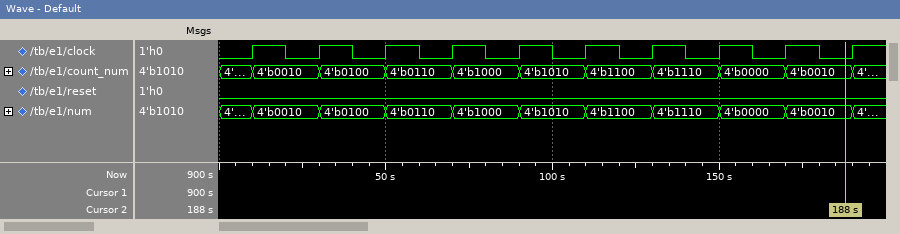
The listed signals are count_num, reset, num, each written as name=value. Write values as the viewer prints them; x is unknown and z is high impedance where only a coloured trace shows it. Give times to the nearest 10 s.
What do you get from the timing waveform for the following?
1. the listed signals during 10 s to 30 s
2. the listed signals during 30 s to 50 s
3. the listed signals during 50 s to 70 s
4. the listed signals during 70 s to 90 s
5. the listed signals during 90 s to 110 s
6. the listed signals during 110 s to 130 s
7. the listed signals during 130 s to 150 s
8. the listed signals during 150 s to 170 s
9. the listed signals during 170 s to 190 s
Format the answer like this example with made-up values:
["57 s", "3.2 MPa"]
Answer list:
["count_num=4'b0010, reset=0, num=4'b0010", "count_num=4'b0100, reset=0, num=4'b0100", "count_num=4'b0110, reset=0, num=4'b0110", "count_num=4'b1000, reset=0, num=4'b1000", "count_num=4'b1010, reset=0, num=4'b1010", "count_num=4'b1100, reset=0, num=4'b1100", "count_num=4'b1110, reset=0, num=4'b1110", "count_num=4'b0000, reset=0, num=4'b0000", "count_num=4'b0010, reset=0, num=4'b0010"]
